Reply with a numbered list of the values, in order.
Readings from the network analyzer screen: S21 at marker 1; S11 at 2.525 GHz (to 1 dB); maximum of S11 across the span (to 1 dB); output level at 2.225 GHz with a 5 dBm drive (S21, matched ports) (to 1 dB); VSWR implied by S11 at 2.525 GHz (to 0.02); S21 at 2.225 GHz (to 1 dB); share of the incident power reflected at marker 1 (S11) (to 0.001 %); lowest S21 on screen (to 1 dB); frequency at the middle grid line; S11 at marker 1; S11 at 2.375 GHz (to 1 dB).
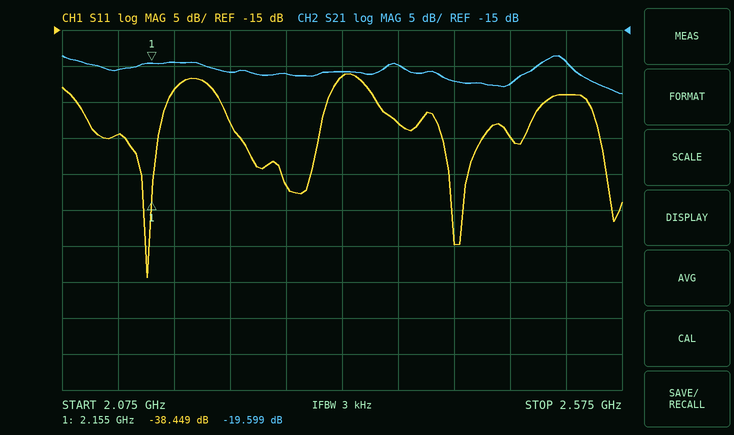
1. -19.599 dB
2. -24 dB
3. -21 dB
4. -16 dBm
5. 1.14
6. -21 dB
7. 0.014 %
8. -24 dB
9. 2.325 GHz
10. -38.449 dB
11. -28 dB
